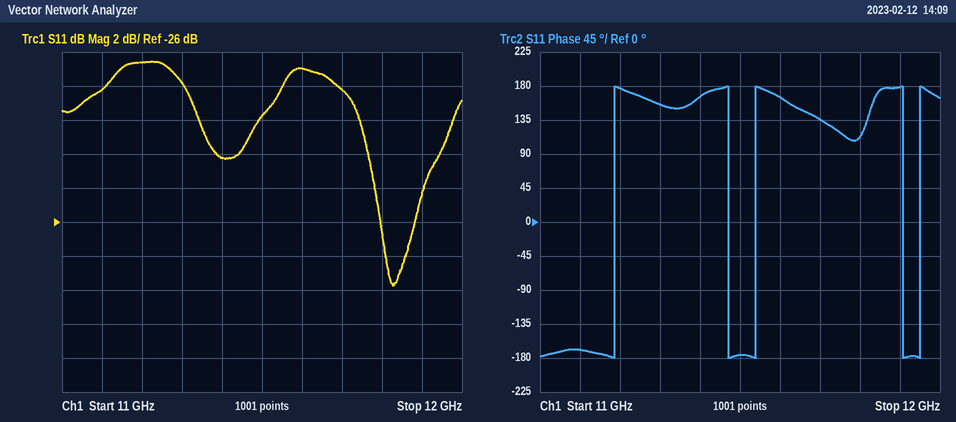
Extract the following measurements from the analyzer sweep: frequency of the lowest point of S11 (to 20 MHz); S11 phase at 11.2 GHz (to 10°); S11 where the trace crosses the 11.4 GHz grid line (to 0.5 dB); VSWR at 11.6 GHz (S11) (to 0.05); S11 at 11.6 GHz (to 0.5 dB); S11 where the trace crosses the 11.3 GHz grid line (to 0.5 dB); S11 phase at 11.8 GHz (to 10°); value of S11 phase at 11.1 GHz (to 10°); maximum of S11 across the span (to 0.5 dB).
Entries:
11.82 GHz
180°
-22.0 dB
1.35
-17.0 dB
-18.0 dB
110°
-170°
-16.5 dB
